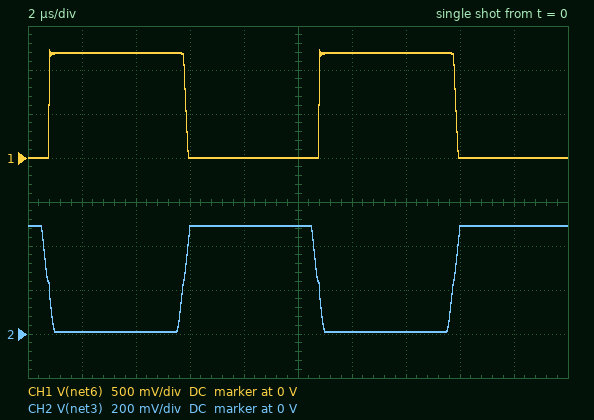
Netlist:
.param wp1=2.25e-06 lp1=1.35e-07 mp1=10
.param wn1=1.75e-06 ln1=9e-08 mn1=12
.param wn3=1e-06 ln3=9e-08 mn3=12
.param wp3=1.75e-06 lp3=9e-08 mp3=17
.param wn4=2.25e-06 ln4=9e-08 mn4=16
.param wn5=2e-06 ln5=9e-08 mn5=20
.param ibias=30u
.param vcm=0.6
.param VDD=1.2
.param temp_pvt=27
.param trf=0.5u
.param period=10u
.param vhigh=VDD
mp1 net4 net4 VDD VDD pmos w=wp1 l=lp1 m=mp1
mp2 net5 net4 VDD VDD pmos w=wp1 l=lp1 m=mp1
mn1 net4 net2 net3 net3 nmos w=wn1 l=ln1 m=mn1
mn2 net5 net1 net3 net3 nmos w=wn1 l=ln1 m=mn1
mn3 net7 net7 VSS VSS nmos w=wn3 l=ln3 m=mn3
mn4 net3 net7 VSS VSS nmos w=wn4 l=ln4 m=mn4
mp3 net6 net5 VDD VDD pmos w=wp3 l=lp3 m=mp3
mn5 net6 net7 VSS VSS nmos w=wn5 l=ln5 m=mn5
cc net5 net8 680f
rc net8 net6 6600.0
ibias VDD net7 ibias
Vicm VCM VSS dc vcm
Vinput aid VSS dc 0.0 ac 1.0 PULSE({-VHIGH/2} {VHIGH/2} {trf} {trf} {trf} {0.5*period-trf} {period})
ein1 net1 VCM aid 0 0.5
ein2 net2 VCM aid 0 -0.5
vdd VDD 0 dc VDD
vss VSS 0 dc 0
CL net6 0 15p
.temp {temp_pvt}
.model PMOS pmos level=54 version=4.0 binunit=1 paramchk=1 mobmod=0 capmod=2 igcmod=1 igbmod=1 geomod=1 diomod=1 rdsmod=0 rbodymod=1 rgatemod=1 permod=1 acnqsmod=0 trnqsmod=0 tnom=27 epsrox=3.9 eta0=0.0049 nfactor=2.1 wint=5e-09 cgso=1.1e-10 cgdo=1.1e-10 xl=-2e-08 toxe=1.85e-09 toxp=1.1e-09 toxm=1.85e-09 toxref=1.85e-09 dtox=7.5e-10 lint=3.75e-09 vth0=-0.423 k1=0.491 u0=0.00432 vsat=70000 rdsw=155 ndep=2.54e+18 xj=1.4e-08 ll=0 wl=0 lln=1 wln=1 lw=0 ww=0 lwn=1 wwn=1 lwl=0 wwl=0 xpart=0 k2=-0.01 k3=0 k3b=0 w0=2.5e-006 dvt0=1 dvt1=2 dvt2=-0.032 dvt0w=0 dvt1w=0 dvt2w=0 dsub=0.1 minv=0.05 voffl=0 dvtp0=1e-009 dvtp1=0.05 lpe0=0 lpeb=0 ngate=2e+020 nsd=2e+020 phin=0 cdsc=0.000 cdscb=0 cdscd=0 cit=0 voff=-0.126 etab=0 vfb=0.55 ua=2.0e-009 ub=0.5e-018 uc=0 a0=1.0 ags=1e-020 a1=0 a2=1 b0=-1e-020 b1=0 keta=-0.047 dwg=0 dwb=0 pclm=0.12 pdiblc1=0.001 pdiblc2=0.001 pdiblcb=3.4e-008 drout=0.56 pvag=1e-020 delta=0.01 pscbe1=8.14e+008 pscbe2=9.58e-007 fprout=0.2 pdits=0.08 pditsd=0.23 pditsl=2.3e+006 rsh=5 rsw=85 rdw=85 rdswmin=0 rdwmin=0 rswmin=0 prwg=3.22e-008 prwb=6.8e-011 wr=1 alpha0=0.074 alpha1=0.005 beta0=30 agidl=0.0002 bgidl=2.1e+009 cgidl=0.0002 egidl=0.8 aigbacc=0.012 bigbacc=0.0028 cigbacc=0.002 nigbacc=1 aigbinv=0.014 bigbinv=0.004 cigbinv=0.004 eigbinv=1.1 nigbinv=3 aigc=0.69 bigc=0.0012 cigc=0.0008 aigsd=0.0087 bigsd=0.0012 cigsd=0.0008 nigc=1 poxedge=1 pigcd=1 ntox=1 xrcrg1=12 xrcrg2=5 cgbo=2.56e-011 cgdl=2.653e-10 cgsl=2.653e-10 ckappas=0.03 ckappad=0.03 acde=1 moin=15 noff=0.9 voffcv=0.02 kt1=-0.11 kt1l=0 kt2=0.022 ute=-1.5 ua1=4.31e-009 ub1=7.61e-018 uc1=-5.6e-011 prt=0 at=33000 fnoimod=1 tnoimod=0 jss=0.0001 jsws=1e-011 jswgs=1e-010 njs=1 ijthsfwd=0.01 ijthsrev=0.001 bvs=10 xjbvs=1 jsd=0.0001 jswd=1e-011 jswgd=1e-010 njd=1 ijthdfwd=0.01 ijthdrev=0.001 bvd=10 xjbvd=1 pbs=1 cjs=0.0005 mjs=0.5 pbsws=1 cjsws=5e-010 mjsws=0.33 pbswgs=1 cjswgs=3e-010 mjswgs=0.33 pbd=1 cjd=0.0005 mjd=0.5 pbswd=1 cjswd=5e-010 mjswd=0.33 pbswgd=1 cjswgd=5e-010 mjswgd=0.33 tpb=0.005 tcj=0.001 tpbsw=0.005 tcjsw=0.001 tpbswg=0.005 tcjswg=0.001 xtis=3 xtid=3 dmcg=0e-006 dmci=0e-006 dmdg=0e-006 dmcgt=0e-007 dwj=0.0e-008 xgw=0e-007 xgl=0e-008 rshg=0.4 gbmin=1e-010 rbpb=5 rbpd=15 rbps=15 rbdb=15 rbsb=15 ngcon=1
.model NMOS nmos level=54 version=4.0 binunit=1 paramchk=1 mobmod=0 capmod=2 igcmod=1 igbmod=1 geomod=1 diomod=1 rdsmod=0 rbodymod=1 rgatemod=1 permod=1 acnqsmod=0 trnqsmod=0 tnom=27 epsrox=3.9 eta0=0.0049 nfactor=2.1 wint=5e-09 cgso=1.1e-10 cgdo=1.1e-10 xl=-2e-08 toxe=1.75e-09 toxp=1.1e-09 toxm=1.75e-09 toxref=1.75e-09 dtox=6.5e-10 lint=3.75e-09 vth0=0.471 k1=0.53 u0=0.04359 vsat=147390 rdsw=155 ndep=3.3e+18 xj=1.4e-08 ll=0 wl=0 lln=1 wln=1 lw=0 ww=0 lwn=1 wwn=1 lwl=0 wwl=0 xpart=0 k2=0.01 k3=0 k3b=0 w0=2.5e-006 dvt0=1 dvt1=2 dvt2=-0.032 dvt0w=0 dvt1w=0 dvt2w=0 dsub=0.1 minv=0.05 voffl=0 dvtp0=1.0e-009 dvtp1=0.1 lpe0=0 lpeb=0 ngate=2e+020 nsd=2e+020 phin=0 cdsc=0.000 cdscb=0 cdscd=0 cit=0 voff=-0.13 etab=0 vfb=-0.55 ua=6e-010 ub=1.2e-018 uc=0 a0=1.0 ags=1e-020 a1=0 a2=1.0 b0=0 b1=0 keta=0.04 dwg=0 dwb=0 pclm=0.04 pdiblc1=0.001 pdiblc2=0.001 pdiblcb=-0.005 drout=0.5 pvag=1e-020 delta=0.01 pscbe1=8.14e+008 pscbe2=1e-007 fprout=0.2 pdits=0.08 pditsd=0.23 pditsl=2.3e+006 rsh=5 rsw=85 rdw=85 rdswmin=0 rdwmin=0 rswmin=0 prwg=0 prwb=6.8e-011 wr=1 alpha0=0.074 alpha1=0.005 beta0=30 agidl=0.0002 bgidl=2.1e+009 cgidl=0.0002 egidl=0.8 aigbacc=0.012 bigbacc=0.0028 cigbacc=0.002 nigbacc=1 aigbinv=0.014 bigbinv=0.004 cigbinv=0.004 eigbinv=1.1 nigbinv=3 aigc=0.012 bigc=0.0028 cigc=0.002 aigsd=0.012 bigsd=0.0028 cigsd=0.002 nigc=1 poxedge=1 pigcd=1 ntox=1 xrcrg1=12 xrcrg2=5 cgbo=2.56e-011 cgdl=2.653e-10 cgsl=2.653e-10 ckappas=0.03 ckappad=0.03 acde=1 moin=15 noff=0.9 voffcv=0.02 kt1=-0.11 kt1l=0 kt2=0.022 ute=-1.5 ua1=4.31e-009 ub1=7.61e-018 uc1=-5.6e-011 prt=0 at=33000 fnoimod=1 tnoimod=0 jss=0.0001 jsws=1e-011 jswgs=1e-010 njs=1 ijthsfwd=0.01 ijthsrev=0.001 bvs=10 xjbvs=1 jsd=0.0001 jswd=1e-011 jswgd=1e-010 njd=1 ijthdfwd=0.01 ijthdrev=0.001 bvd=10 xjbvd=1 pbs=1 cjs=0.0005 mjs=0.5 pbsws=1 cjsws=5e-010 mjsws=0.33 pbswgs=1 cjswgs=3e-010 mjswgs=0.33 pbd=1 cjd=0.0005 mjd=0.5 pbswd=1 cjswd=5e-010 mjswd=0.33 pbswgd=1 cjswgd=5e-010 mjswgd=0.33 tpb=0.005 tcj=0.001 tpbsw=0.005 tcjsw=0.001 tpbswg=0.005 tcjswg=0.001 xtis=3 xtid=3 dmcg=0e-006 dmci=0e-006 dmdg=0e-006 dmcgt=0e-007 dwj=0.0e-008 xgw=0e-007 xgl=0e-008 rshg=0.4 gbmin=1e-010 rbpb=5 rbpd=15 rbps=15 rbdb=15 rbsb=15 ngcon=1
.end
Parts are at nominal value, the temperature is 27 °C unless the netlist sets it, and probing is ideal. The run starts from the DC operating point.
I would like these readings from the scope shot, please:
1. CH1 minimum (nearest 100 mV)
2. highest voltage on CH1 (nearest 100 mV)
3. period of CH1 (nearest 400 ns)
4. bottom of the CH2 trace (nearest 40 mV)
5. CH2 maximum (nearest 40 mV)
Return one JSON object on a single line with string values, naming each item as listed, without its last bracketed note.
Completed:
{"CH1 minimum": "0 V", "highest voltage on CH1": "1.2 V", "period of CH1": "10.0 µs", "bottom of the CH2 trace": "0 V", "CH2 maximum": "480 mV"}
